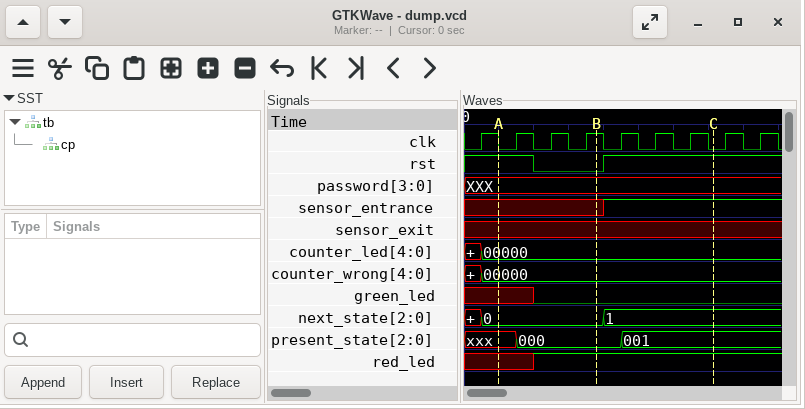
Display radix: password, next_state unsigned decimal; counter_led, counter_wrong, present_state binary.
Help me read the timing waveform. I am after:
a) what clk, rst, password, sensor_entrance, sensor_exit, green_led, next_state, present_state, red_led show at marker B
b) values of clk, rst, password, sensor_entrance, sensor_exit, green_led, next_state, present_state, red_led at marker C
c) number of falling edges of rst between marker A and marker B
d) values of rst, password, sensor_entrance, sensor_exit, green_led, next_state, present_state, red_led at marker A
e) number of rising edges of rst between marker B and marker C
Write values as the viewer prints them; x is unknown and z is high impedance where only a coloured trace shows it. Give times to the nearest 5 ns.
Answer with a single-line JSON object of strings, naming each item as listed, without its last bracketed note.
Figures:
{"what clk, rst, password, sensor_entrance, sensor_exit, green_led, next_state, present_state, red_led show at marker B": "clk=1, rst=0, password=XXX, sensor_entrance=x, sensor_exit=x, green_led=0, next_state=0, present_state=000, red_led=1", "values of clk, rst, password, sensor_entrance, sensor_exit, green_led, next_state, present_state, red_led at marker C": "clk=0, rst=1, password=XXX, sensor_entrance=1, sensor_exit=x, green_led=0, next_state=1, present_state=001, red_led=1", "number of falling edges of rst between marker A and marker B": "1", "values of rst, password, sensor_entrance, sensor_exit, green_led, next_state, present_state, red_led at marker A": "rst=1, password=XXX, sensor_entrance=x, sensor_exit=x, green_led=x, next_state=0, present_state=xxx, red_led=x", "number of rising edges of rst between marker B and marker C": "1"}
